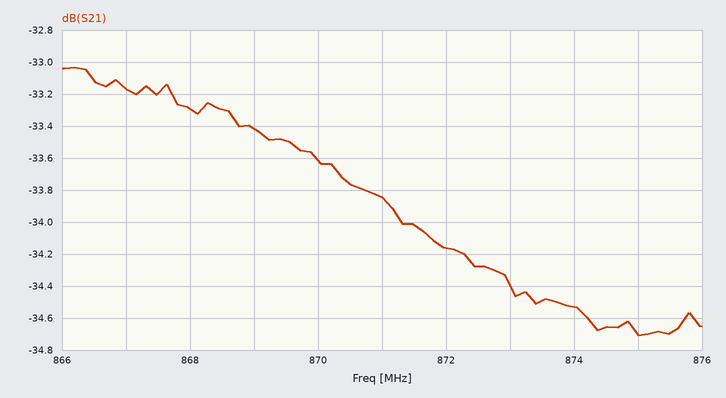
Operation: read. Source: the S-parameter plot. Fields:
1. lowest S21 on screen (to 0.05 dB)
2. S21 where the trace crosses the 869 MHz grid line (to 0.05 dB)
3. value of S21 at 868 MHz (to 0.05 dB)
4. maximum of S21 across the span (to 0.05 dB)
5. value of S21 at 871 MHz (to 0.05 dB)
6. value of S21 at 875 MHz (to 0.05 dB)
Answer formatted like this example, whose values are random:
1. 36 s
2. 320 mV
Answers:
1. -34.70 dB
2. -33.40 dB
3. -33.30 dB
4. -33.05 dB
5. -33.85 dB
6. -34.70 dB
